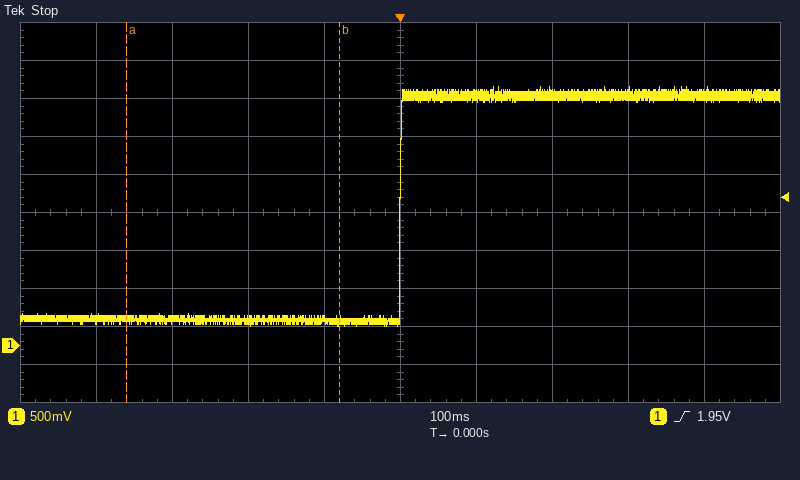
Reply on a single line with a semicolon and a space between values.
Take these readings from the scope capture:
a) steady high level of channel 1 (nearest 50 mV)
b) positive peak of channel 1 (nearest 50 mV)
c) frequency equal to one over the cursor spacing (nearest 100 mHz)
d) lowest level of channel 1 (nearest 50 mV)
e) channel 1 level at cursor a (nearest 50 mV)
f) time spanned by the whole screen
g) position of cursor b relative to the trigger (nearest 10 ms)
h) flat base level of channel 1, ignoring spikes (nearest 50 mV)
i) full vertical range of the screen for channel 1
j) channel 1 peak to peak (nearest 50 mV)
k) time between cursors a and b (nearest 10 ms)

3.30 V; 3.40 V; 3.6 Hz; 250 mV; 350 mV; 1 s; -80 ms; 350 mV; 5 V; 3.15 V; 280 ms
